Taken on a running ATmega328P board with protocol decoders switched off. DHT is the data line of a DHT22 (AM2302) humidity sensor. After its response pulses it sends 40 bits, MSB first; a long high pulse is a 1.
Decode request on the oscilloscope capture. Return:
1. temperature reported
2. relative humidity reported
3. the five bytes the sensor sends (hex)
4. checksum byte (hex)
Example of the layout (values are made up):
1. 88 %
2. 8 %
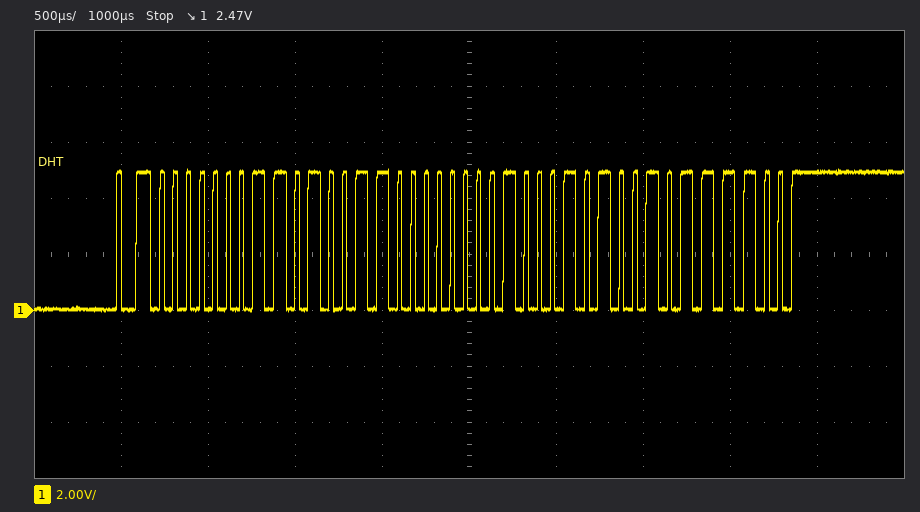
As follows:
1. 27.6 °C
2. 42.2 %
3. 01 A6 01 14 BC
4. 0xBC
